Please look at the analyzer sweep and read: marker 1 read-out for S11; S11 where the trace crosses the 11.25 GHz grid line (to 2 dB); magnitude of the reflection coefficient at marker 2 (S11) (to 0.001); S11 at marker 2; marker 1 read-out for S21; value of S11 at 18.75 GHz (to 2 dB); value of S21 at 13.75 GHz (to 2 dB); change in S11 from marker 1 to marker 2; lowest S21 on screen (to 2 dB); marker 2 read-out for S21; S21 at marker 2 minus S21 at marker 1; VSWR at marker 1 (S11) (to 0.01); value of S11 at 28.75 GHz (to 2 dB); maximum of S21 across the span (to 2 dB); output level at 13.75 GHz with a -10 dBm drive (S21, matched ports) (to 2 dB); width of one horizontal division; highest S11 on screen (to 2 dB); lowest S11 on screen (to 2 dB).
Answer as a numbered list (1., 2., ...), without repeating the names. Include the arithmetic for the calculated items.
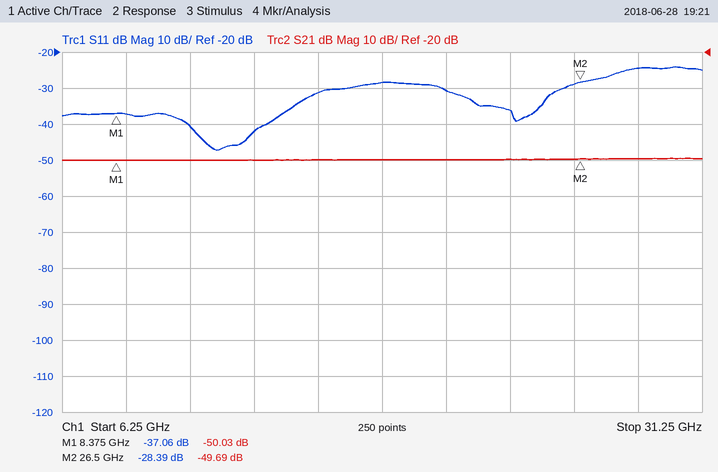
1. -37.06 dB
2. -40 dB
3. 10^(-28.39/20) ≈ 0.038
4. -28.39 dB
5. -50.03 dB
6. -28 dB
7. -50 dB
8. -28.39 − (-37.06) = 8.67 dB
9. -50 dB
10. -49.69 dB
11. -49.69 − (-50.03) = 0.34 dB
12. (1 + 0.0140)/(1 − 0.0140) ≈ 1.03
13. -24 dB
14. -50 dB
15. -10 dBm + (-50 dB) = -60 dBm
16. 2.5 GHz
17. -24 dB
18. -48 dB
